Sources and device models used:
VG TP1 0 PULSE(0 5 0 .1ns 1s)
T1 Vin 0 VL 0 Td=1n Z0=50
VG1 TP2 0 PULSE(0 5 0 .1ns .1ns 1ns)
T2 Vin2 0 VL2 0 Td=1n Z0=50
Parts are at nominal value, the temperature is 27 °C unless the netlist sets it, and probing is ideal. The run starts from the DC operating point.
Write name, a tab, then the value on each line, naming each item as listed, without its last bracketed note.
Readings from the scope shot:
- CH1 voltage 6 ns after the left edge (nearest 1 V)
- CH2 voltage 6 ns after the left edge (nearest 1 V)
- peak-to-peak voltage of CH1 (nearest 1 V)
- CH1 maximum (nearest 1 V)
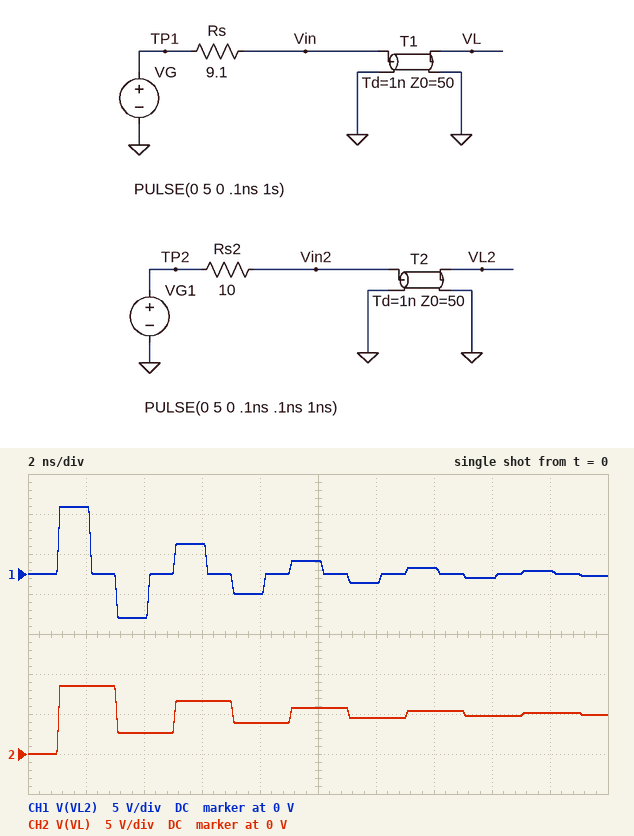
CH1 voltage 6 ns after the left edge	4 V
CH2 voltage 6 ns after the left edge	7 V
peak-to-peak voltage of CH1	14 V
CH1 maximum	8 V
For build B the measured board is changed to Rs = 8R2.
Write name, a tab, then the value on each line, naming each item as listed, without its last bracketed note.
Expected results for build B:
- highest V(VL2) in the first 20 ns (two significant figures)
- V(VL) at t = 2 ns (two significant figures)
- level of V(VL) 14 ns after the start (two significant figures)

highest V(VL2) in the first 20 ns	8.3 V
V(VL) at t = 2 ns	8.6 V
level of V(VL) 14 ns after the start	5.5 V
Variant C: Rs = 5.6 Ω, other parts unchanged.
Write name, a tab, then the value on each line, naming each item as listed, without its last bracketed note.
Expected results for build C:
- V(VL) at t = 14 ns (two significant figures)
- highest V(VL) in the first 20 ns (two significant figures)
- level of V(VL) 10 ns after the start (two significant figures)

V(VL) at t = 14 ns	6.0 V
highest V(VL) in the first 20 ns	9.0 V
level of V(VL) 10 ns after the start	6.6 V
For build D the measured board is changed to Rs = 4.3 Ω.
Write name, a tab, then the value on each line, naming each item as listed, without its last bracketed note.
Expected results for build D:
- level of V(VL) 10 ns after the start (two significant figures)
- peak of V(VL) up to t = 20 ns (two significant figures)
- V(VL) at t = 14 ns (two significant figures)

level of V(VL) 10 ns after the start	7.1 V
peak of V(VL) up to t = 20 ns	9.2 V
V(VL) at t = 14 ns	6.5 V
